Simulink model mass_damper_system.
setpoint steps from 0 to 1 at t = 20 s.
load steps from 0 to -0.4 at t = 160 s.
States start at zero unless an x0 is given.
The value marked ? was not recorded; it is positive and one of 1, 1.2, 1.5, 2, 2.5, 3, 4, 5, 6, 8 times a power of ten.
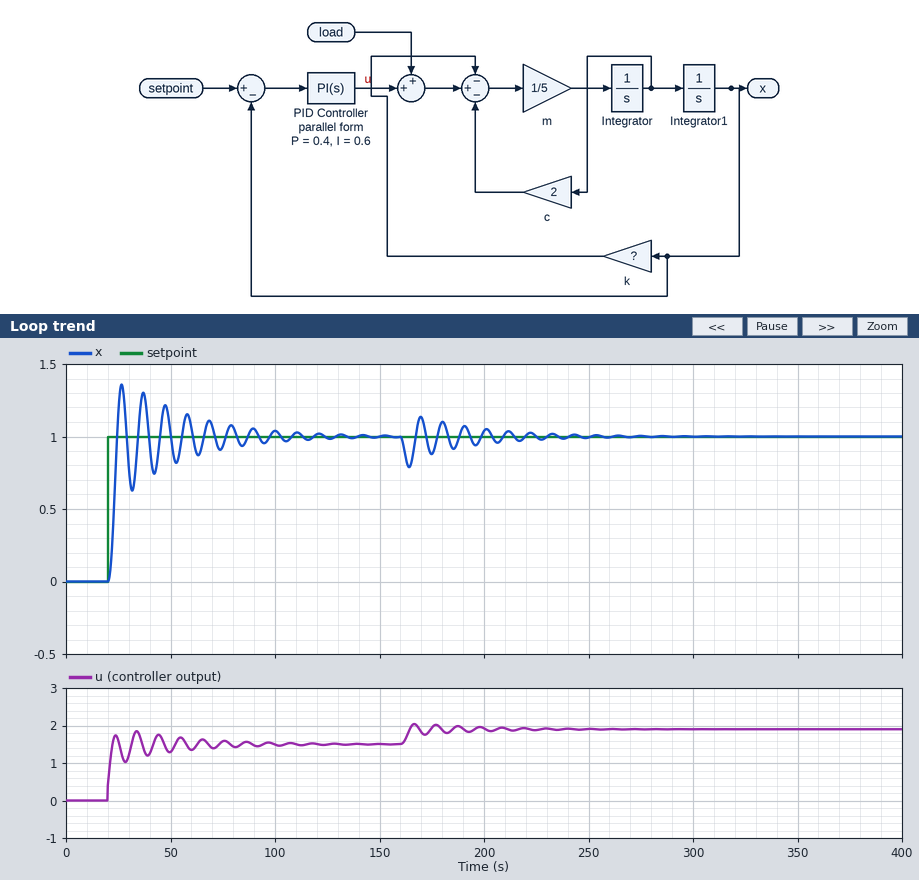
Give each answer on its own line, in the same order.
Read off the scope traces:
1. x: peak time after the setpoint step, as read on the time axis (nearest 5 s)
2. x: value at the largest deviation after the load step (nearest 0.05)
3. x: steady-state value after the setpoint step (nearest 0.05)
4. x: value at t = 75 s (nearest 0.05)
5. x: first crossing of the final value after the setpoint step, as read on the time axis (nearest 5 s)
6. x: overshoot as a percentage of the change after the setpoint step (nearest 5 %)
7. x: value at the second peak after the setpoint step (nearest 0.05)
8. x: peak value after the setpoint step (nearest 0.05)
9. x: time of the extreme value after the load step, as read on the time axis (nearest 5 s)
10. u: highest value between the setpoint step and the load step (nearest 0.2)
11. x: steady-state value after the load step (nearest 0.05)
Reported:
25 s
0.80
1.00
0.95
25 s
35 %
1.30
1.35
165 s
1.8
1.00
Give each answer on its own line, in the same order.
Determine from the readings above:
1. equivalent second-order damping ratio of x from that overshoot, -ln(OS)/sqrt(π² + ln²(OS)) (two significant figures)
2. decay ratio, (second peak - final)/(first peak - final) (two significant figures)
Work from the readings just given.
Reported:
0.32
0.86
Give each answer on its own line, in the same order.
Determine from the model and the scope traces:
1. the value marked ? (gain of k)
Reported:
1.5
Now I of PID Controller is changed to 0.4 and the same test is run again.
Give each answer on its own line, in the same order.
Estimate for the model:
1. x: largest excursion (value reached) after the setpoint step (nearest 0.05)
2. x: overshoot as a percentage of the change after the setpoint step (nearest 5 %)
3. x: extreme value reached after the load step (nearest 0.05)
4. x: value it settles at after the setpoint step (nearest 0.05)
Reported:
1.10
10 %
0.75
1.00
